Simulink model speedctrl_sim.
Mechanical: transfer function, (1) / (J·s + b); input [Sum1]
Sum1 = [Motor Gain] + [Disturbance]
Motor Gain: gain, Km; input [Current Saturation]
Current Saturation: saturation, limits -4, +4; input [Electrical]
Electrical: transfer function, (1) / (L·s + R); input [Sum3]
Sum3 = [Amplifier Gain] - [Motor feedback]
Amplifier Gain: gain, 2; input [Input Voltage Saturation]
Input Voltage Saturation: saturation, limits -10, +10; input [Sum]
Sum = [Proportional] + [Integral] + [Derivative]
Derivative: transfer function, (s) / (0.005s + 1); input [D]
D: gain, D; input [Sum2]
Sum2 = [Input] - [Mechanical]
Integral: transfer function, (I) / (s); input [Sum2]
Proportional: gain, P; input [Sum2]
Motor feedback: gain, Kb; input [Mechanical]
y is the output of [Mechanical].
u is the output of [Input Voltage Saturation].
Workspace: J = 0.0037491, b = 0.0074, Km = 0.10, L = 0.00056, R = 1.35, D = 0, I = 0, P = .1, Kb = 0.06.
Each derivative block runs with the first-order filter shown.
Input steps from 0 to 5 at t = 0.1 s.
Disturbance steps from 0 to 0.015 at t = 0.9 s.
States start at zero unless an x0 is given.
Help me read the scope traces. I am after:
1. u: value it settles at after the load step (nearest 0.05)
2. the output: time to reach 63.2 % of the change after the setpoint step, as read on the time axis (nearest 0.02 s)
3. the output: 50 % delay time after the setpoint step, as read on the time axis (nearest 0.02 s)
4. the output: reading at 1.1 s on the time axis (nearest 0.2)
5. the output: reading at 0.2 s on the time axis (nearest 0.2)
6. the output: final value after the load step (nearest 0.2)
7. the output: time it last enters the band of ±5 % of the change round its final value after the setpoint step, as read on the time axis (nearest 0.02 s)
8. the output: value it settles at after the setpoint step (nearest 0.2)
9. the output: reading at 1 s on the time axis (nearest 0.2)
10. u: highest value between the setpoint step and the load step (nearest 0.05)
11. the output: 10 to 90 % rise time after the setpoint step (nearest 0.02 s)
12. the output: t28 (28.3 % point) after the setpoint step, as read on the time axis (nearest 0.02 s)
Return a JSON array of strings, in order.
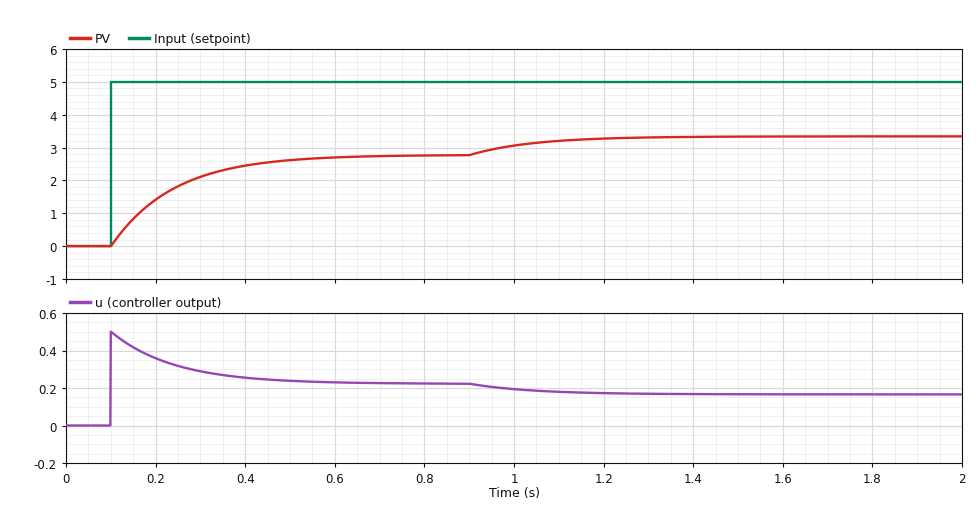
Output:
["0.15", "0.24 s", "0.20 s", "3.2", "1.4", "3.4", "0.52 s", "2.8", "3.0", "0.50", "0.30 s", "0.14 s"]
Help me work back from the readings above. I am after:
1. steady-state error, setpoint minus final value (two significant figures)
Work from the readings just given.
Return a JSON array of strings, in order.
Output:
["2.2"]
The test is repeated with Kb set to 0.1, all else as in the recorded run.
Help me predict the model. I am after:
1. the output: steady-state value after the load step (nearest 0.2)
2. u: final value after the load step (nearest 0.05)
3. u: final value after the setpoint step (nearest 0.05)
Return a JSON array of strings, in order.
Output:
["3.0", "0.20", "0.25"]
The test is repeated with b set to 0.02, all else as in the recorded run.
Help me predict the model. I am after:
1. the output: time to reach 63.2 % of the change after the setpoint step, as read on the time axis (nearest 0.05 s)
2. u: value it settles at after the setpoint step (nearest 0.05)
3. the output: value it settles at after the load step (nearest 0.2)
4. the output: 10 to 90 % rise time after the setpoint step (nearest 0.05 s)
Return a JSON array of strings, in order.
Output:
["0.20 s", "0.30", "2.2", "0.20 s"]
